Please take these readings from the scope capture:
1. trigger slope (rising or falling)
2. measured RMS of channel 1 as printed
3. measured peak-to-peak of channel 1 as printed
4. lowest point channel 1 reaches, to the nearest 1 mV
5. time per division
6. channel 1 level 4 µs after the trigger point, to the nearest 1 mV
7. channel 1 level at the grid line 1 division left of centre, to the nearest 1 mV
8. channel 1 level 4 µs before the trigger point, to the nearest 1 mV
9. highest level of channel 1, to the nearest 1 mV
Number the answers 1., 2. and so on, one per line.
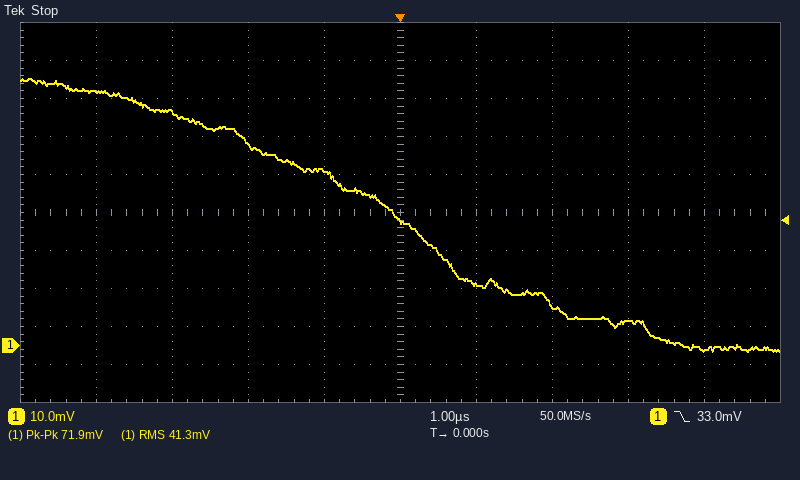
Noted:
1. falling
2. 41.3 mV
3. 71.9 mV
4. -2 mV
5. 1 µs
6. -1 mV
7. 46 mV
8. 67 mV
9. 70 mV
